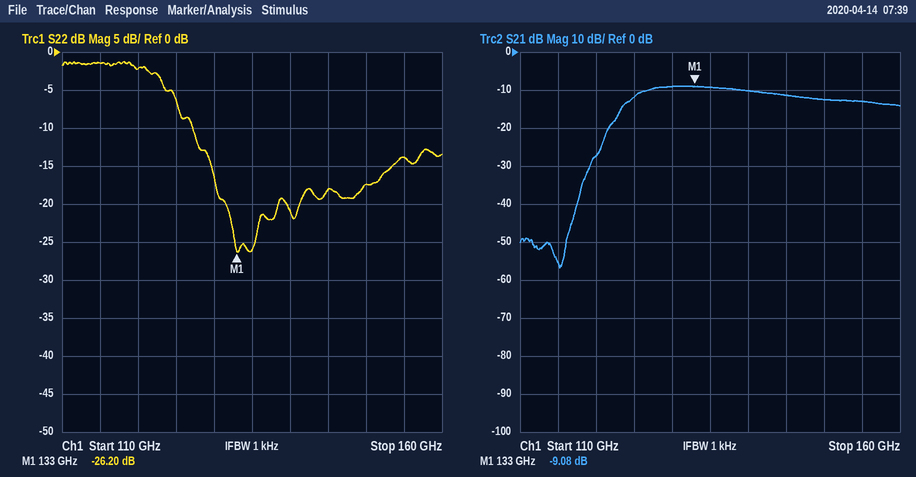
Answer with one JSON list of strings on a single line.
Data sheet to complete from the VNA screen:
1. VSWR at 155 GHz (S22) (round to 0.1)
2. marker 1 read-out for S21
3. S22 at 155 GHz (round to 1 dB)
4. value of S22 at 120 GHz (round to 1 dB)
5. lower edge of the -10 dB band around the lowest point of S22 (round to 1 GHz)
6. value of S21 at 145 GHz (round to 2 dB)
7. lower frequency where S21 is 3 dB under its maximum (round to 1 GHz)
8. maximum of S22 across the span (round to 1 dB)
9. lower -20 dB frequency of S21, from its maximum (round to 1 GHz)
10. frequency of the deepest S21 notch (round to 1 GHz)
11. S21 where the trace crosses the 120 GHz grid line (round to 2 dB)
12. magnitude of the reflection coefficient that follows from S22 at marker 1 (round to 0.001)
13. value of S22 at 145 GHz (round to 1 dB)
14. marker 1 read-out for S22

["1.5", "-9.08 dB", "-14 dB", "-2 dB", "127 GHz", "-12 dB", "125 GHz", "-1 dB", "119 GHz", "115 GHz", "-28 dB", "0.049", "-18 dB", "-26.20 dB"]
